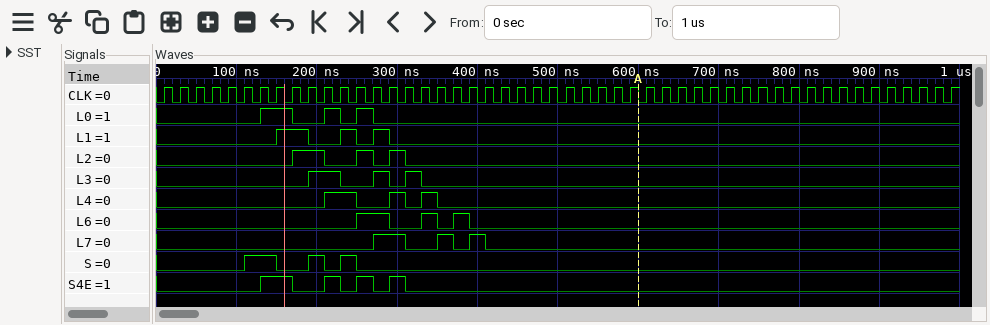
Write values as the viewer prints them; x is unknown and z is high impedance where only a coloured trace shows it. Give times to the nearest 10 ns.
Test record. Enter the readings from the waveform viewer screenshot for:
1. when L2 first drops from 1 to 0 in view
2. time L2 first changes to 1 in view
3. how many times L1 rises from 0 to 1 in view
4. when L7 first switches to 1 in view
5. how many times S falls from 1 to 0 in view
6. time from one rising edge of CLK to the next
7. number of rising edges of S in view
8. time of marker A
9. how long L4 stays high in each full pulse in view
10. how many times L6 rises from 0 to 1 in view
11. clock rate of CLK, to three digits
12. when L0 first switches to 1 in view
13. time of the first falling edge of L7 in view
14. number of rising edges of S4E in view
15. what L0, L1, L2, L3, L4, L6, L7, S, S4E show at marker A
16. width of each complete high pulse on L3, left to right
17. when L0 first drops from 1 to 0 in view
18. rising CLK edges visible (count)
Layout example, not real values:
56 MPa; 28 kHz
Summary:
210 ns; 170 ns; 3; 270 ns; 3; 20 ns; 3; 600 ns; 40 ns, 20 ns, 20 ns; 3; 50.0 MHz; 130 ns; 310 ns; 4; L0=0, L1=0, L2=0, L3=0, L4=0, L6=0, L7=0, S=0, S4E=0; 40 ns, 20 ns, 20 ns; 170 ns; 50
